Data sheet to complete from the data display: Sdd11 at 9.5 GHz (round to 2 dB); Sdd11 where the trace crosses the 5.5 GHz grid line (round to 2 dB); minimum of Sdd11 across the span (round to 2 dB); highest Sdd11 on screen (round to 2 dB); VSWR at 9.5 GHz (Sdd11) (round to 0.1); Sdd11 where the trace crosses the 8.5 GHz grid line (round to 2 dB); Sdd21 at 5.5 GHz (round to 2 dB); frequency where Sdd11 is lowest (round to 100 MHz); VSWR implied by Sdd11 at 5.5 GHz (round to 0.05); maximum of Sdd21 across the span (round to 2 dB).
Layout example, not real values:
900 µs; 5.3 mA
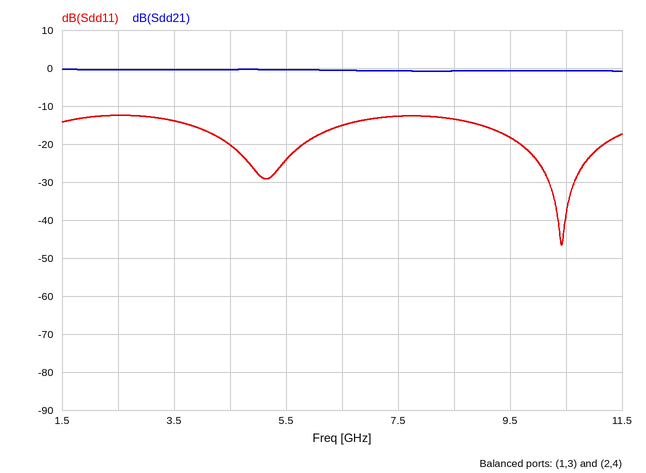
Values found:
-18 dB; -24 dB; -46 dB; -12 dB; 1.3; -14 dB; 0 dB; 10.4 GHz; 1.15; 0 dB
